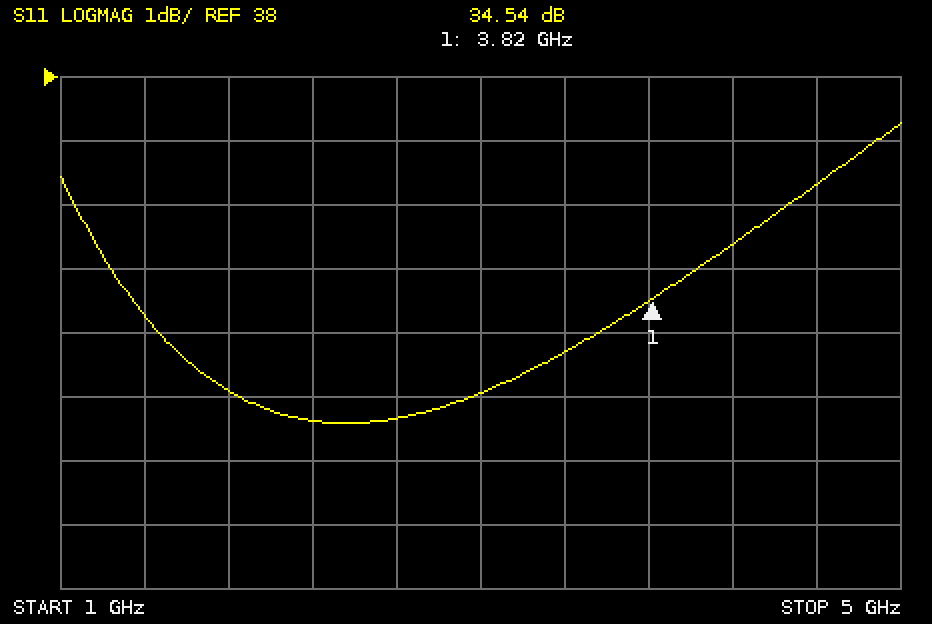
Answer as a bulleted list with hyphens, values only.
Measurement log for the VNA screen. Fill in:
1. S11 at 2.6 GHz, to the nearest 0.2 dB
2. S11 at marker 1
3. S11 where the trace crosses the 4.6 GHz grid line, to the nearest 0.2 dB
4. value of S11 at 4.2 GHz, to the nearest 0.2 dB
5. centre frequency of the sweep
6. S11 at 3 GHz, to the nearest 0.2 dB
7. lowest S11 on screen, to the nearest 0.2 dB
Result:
- 32.6 dB
- 34.54 dB
- 36.4 dB
- 35.4 dB
- 3 GHz
- 33.0 dB
- 32.6 dB
